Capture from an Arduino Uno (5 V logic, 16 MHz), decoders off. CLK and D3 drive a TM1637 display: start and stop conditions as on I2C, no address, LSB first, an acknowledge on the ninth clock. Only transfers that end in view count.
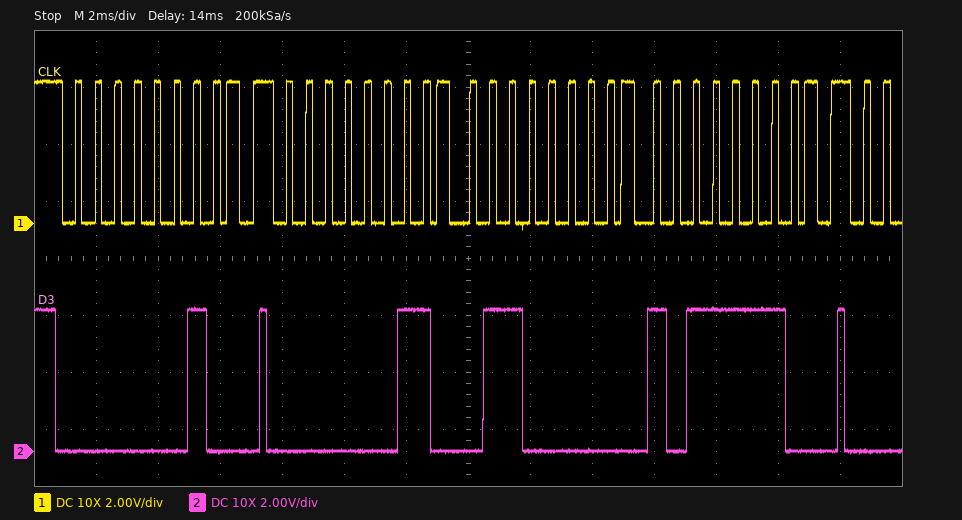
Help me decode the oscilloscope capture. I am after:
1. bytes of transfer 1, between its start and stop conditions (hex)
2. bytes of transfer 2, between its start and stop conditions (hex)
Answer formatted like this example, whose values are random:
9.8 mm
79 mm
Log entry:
40
C0 06 7D
